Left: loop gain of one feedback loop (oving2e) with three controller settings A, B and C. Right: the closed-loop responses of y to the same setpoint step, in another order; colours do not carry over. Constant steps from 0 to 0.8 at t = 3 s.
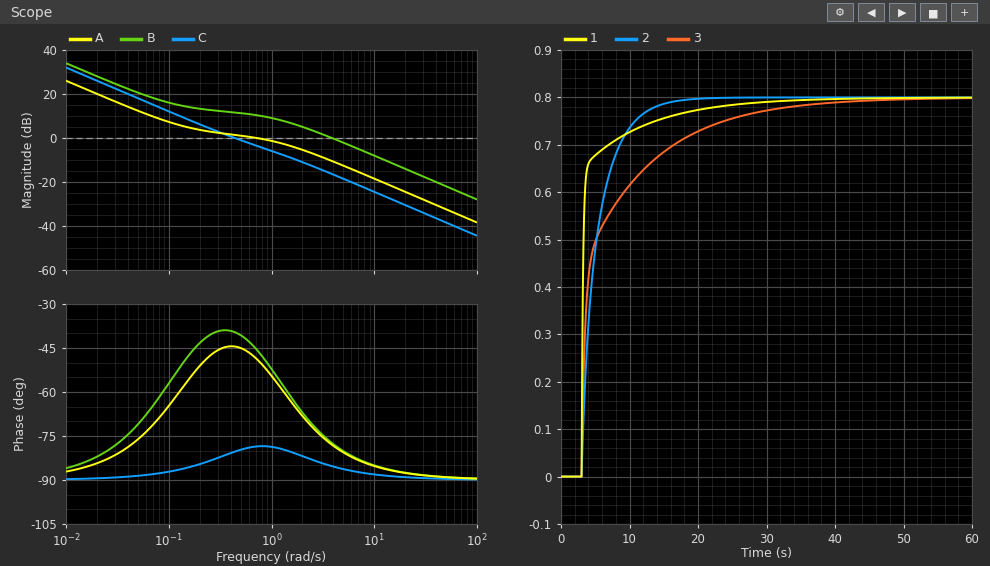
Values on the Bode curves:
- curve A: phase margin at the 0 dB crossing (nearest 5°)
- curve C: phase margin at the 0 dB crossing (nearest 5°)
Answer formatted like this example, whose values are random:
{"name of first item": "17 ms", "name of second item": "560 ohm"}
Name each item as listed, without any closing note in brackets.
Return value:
{"curve A: phase margin at the 0 dB crossing": "130°", "curve C: phase margin at the 0 dB crossing": "100°"}
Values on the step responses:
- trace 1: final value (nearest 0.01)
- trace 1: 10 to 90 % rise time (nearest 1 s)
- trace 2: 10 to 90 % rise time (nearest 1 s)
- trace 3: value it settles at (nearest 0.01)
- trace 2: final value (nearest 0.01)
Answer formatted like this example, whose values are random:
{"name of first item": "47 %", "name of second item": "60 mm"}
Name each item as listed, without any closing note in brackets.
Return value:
{"trace 1: final value": "0.80", "trace 1: 10 to 90 % rise time": "6 s", "trace 2: 10 to 90 % rise time": "6 s", "trace 3: value it settles at": "0.80", "trace 2: final value": "0.80"}
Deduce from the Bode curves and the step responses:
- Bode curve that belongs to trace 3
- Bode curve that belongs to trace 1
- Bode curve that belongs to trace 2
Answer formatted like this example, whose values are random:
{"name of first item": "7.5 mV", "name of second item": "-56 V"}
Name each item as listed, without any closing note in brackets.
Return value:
{"Bode curve that belongs to trace 3": "A", "Bode curve that belongs to trace 1": "B", "Bode curve that belongs to trace 2": "C"}
